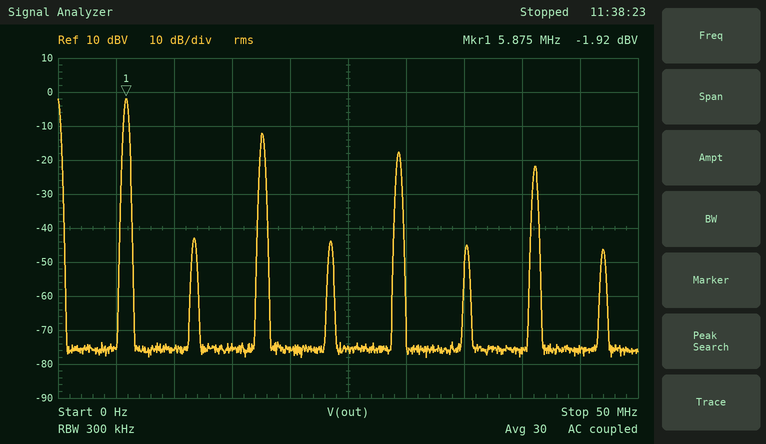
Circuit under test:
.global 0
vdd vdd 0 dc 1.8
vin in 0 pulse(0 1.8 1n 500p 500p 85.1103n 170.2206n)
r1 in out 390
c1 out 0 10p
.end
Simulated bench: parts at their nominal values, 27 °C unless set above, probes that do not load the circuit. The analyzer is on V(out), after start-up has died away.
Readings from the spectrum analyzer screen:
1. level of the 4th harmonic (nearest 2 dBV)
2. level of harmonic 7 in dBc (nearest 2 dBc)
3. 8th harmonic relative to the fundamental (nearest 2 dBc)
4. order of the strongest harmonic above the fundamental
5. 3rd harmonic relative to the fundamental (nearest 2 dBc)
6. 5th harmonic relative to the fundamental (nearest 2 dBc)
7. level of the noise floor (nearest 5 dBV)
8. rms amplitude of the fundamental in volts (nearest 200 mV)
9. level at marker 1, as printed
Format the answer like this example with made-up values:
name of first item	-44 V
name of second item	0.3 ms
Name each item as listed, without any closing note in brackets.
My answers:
level of the 4th harmonic	-44 dBV
level of harmonic 7 in dBc	-20 dBc
8th harmonic relative to the fundamental	-44 dBc
order of the strongest harmonic above the fundamental	3
3rd harmonic relative to the fundamental	-10 dBc
5th harmonic relative to the fundamental	-16 dBc
level of the noise floor	-75 dBV
rms amplitude of the fundamental in volts	800 mV
level at marker 1, as printed	-1.92 dBV
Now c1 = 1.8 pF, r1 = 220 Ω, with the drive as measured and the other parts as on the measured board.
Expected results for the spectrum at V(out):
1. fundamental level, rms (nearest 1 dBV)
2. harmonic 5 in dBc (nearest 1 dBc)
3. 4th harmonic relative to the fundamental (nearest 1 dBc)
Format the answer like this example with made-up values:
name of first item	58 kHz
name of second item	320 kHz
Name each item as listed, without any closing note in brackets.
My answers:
fundamental level, rms	-2 dBV
harmonic 5 in dBc	-14 dBc
4th harmonic relative to the fundamental	-41 dBc
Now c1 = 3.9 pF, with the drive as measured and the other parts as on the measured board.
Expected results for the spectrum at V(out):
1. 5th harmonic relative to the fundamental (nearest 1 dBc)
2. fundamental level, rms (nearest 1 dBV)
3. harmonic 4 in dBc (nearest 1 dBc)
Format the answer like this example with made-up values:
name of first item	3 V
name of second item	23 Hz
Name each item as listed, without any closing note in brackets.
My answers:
5th harmonic relative to the fundamental	-14 dBc
fundamental level, rms	-2 dBV
harmonic 4 in dBc	-41 dBc
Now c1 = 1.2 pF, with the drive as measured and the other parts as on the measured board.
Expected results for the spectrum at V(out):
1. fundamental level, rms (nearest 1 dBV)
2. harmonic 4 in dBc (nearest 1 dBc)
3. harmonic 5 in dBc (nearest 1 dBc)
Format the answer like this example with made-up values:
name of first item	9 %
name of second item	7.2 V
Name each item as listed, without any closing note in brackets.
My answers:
fundamental level, rms	-2 dBV
harmonic 4 in dBc	-41 dBc
harmonic 5 in dBc	-14 dBc
